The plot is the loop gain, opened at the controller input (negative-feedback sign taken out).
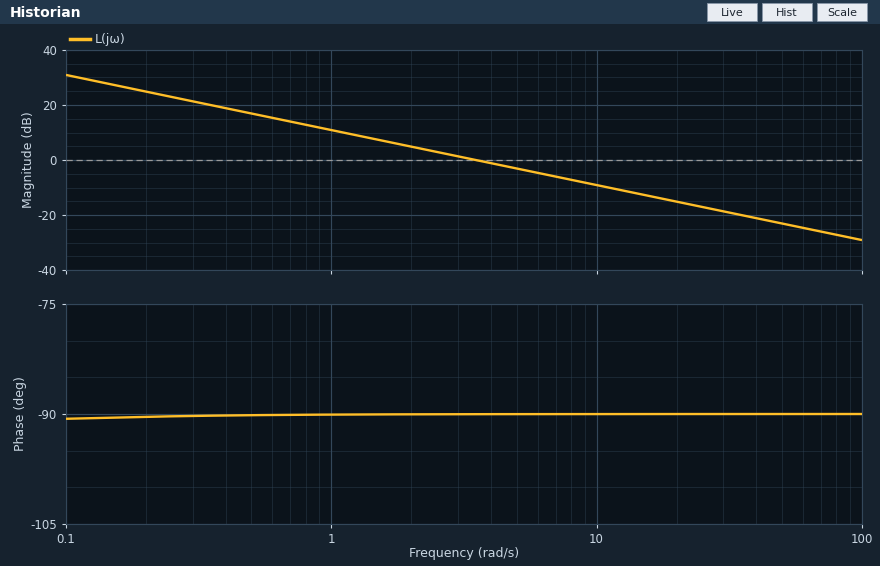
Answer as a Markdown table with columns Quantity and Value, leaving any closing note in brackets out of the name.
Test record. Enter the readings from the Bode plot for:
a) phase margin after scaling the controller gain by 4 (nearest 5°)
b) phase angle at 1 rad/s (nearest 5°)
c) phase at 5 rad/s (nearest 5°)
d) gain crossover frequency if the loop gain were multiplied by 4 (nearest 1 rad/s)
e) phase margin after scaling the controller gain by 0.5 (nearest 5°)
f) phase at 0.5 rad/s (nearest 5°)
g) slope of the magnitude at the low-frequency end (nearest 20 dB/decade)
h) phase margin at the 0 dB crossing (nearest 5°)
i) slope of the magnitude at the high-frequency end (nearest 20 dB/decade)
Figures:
| Quantity | Value |
|---|---|
| phase margin after scaling the controller gain by 4 | 90° |
| phase angle at 1 rad/s | -90° |
| phase at 5 rad/s | -90° |
| gain crossover frequency if the loop gain were multiplied by 4 | 14 rad/s |
| phase margin after scaling the controller gain by 0.5 | 90° |
| phase at 0.5 rad/s | -90° |
| slope of the magnitude at the low-frequency end | -20 dB/decade |
| phase margin at the 0 dB crossing | 90° |
| slope of the magnitude at the high-frequency end | -20 dB/decade |
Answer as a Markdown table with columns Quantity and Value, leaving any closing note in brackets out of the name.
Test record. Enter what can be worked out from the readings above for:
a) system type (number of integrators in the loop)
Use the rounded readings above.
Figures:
| Quantity | Value |
|---|---|
| system type | 1 |
